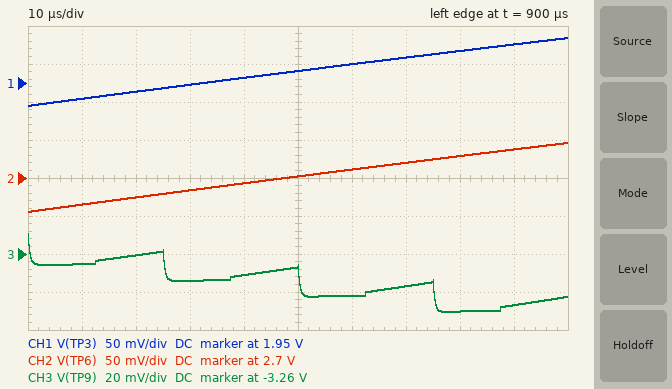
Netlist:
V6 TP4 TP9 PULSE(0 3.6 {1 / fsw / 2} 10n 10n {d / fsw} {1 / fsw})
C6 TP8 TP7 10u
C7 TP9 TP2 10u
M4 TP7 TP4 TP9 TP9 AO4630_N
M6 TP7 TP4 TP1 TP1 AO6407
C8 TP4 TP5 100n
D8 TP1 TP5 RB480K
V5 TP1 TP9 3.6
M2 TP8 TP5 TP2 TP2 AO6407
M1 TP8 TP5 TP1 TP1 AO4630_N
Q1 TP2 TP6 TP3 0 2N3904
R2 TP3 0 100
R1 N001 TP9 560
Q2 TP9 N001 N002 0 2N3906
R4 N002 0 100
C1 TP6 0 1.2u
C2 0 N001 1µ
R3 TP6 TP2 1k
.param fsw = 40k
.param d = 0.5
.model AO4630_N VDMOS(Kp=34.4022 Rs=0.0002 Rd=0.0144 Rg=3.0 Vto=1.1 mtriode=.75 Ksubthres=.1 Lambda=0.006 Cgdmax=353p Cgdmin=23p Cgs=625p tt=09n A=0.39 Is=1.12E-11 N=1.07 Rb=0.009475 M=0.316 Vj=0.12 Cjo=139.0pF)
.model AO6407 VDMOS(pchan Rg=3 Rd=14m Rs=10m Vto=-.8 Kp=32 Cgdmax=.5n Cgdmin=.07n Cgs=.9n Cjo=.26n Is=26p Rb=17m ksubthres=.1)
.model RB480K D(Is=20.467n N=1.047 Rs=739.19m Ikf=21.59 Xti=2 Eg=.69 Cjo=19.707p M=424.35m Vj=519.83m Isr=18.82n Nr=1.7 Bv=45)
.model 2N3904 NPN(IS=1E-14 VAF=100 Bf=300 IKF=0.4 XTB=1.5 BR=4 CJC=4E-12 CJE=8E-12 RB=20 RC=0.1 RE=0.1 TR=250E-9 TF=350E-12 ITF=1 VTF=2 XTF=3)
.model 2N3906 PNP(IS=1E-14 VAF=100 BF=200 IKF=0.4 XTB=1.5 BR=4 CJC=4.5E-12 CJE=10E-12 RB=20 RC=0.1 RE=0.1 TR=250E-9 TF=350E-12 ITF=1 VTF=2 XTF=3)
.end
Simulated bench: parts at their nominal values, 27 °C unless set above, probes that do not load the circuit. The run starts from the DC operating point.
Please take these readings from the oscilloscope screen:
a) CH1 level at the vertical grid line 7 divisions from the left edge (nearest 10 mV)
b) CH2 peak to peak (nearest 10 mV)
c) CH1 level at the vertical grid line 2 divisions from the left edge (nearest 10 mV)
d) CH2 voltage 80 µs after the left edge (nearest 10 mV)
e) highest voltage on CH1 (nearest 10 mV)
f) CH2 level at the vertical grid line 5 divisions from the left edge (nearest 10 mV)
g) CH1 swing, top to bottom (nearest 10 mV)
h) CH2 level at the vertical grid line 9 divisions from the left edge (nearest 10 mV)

1.98 V
90 mV
1.94 V
2.73 V
2.01 V
2.70 V
90 mV
2.74 V
